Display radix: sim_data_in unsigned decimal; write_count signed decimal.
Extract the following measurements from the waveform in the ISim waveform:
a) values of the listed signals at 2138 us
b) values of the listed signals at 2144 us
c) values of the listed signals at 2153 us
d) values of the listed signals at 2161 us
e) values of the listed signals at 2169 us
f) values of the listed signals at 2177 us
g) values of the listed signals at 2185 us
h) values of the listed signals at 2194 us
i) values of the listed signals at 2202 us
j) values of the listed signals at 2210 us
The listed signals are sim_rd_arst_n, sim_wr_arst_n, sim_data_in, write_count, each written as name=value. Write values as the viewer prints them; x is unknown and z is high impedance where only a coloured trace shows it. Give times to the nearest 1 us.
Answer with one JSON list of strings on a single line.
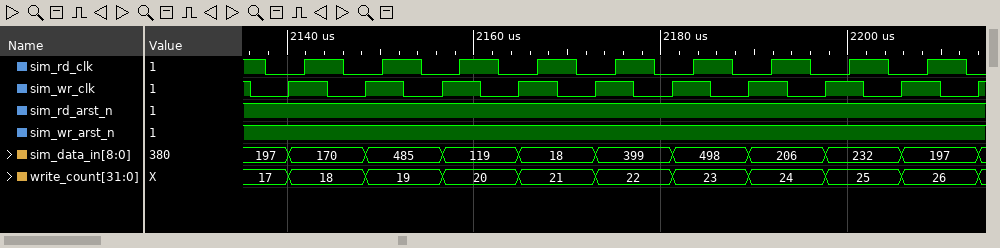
["sim_rd_arst_n=1, sim_wr_arst_n=1, sim_data_in=197, write_count=17", "sim_rd_arst_n=1, sim_wr_arst_n=1, sim_data_in=170, write_count=18", "sim_rd_arst_n=1, sim_wr_arst_n=1, sim_data_in=485, write_count=19", "sim_rd_arst_n=1, sim_wr_arst_n=1, sim_data_in=119, write_count=20", "sim_rd_arst_n=1, sim_wr_arst_n=1, sim_data_in=18, write_count=21", "sim_rd_arst_n=1, sim_wr_arst_n=1, sim_data_in=399, write_count=22", "sim_rd_arst_n=1, sim_wr_arst_n=1, sim_data_in=498, write_count=23", "sim_rd_arst_n=1, sim_wr_arst_n=1, sim_data_in=206, write_count=24", "sim_rd_arst_n=1, sim_wr_arst_n=1, sim_data_in=232, write_count=25", "sim_rd_arst_n=1, sim_wr_arst_n=1, sim_data_in=197, write_count=26"]
